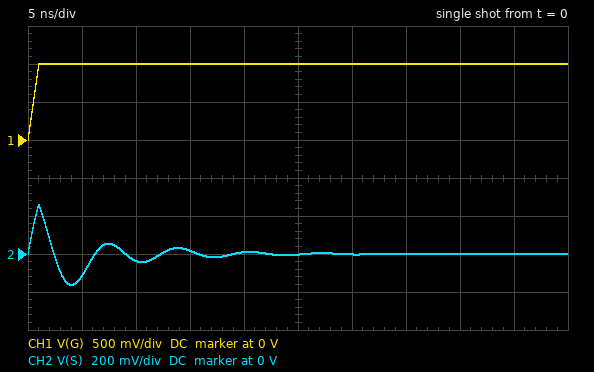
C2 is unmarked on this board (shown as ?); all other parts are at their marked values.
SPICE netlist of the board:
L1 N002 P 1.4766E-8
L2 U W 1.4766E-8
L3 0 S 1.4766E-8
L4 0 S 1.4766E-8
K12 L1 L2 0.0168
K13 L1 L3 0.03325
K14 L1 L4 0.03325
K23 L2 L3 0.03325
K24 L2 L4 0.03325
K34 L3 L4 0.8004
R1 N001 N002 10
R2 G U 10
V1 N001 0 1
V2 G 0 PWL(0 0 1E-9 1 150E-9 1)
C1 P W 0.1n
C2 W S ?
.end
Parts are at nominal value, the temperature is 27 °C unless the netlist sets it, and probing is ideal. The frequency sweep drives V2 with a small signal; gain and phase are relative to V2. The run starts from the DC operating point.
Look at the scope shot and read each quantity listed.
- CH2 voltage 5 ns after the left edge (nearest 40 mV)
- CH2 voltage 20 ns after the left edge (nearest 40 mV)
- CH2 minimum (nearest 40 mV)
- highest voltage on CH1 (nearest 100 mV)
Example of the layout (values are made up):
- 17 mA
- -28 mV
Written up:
- -120 mV
- 0 V
- -160 mV
- 1.0 V
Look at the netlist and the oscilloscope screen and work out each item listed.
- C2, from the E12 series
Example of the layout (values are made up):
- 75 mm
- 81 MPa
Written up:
- 68 pF
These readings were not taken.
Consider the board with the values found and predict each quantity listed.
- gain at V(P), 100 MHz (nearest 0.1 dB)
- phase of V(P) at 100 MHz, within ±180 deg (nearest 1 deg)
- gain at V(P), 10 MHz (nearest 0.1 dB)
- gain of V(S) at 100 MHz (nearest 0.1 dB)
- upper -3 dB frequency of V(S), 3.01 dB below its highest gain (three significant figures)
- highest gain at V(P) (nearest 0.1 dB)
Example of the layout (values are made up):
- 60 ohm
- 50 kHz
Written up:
- -4.4 dB
- 8 deg
- -24.0 dB
- -11.1 dB
- 190 MHz
- -4.2 dB
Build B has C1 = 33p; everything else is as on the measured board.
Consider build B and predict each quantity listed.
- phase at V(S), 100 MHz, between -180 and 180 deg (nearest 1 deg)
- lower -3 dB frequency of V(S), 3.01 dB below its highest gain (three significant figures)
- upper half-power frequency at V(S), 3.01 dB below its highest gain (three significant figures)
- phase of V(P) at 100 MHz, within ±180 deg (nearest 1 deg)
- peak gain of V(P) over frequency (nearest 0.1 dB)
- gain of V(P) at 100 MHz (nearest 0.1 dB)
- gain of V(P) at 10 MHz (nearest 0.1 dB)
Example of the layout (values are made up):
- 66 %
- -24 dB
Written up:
- 105 deg
- 100 MHz
- 224 MHz
- 45 deg
- -6.0 dB
- -9.1 dB
- -33.6 dB
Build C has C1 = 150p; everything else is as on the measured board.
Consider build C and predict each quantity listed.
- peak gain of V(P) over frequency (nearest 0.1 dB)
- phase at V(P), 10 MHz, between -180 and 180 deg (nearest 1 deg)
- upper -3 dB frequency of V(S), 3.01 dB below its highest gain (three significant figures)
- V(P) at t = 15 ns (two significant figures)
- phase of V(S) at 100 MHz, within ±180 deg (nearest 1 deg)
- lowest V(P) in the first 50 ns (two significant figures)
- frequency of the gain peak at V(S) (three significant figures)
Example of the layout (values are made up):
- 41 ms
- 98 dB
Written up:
- -3.4 dB
- 82 deg
- 181 MHz
- 970 mV
- 127 deg
- 940 mV
- 150 MHz
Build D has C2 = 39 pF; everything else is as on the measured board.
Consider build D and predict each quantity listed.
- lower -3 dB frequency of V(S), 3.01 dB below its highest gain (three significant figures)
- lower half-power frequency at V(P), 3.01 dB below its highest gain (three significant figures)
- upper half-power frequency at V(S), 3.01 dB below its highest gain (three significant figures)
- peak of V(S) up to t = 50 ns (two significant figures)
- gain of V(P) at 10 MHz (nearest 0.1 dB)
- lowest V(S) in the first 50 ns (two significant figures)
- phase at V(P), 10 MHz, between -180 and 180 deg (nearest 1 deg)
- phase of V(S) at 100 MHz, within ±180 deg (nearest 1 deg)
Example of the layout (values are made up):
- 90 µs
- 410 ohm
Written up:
- 176 MHz
- 81.5 MHz
- 223 MHz
- 240 mV
- -24.0 dB
- -180 mV
- 87 deg
- 125 deg
